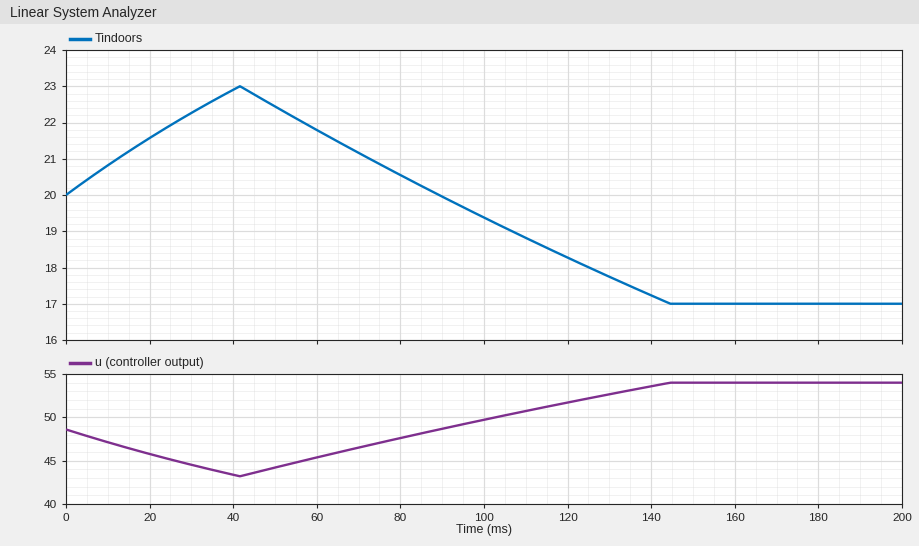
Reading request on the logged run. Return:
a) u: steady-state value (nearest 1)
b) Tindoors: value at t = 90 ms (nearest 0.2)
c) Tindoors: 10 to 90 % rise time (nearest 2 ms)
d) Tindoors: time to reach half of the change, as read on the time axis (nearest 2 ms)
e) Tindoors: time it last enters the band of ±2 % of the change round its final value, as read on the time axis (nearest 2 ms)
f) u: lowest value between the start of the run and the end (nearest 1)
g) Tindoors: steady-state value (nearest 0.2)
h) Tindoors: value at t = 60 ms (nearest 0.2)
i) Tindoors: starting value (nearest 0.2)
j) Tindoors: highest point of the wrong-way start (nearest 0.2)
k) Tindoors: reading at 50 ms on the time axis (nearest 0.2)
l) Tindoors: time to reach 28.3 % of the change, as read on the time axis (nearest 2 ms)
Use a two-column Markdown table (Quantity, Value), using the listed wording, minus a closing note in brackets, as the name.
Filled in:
| Quantity | Value |
|---|---|
| u: steady-state value | 54 |
| Tindoors: value at t = 90 ms | 20.0 |
| Tindoors: 10 to 90 % rise time | 44 ms |
| Tindoors: time to reach half of the change, as read on the time axis | 116 ms |
| Tindoors: time it last enters the band of ±2 % of the change round its final value, as read on the time axis | 144 ms |
| u: lowest value between the start of the run and the end | 43 |
| Tindoors: steady-state value | 17.0 |
| Tindoors: value at t = 60 ms | 21.8 |
| Tindoors: starting value | 20.0 |
| Tindoors: highest point of the wrong-way start | 23.0 |
| Tindoors: reading at 50 ms on the time axis | 22.4 |
| Tindoors: time to reach 28.3 % of the change, as read on the time axis | 104 ms |
